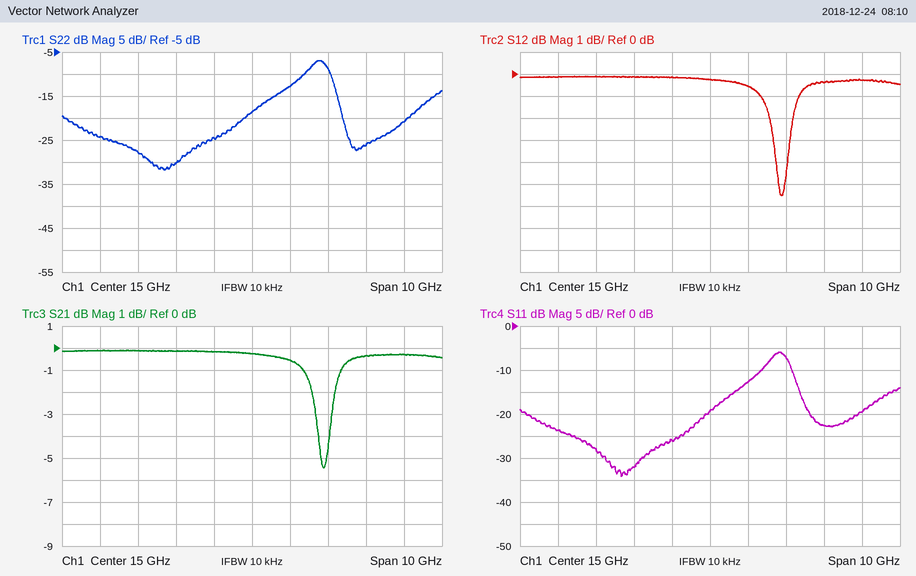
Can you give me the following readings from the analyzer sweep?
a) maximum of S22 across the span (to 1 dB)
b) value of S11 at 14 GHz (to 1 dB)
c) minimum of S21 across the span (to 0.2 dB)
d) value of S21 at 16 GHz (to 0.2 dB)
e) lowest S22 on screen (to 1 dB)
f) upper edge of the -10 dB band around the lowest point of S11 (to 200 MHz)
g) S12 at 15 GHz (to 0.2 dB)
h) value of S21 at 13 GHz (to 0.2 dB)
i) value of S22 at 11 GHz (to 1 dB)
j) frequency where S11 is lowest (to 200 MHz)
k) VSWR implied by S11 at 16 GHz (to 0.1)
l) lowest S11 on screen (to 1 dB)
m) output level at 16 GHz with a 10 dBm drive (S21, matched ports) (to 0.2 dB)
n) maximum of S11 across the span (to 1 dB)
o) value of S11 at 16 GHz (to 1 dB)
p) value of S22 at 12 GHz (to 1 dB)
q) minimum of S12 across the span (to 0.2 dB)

-7 dB
-26 dB
-5.4 dB
-0.6 dB
-32 dB
16.4 GHz
-0.2 dB
-0.2 dB
-24 dB
12.6 GHz
1.6
-34 dB
9.4 dBm
-6 dB
-13 dB
-28 dB
-5.6 dB
